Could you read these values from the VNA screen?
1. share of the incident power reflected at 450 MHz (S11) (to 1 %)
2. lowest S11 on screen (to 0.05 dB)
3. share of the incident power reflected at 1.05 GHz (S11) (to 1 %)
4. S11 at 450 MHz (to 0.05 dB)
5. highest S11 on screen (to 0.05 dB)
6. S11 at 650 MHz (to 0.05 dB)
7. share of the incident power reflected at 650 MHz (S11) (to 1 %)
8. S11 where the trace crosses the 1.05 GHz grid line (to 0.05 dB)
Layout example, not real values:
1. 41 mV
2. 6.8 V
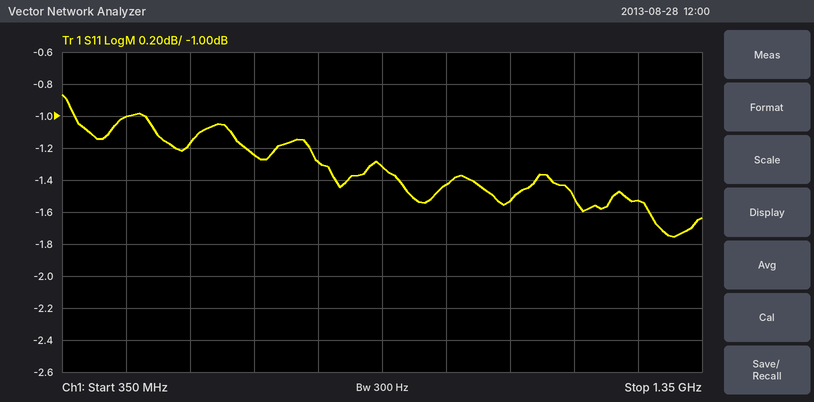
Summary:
1. 79 %
2. -1.75 dB
3. 70 %
4. -1.00 dB
5. -0.85 dB
6. -1.25 dB
7. 75 %
8. -1.55 dB
